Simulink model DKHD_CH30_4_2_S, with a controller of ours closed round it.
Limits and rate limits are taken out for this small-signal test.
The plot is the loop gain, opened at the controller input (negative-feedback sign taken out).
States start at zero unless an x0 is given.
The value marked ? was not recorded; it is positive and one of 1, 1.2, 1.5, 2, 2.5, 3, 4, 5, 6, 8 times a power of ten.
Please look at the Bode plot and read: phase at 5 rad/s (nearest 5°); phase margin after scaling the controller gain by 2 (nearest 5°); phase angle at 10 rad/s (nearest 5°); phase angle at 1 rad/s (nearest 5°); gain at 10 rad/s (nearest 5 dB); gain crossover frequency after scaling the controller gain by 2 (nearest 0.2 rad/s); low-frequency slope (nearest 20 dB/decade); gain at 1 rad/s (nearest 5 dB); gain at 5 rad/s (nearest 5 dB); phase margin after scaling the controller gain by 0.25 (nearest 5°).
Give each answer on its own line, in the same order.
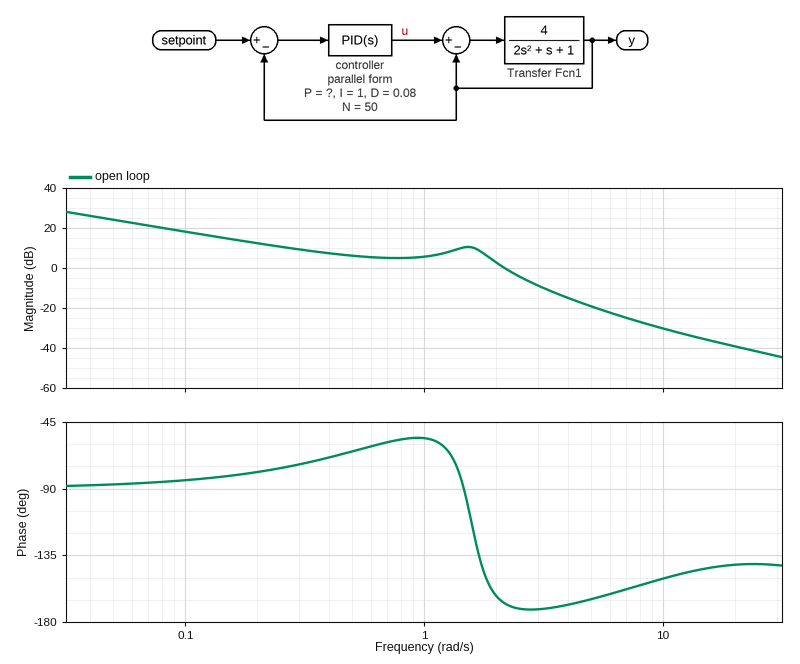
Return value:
-165°
10°
-150°
-55°
-30 dB
2.6 rad/s
-20 dB/decade
5 dB
-20 dB
100°
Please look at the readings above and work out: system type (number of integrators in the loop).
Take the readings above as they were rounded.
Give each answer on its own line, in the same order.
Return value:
1
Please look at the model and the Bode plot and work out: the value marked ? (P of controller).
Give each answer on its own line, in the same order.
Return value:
1.2
